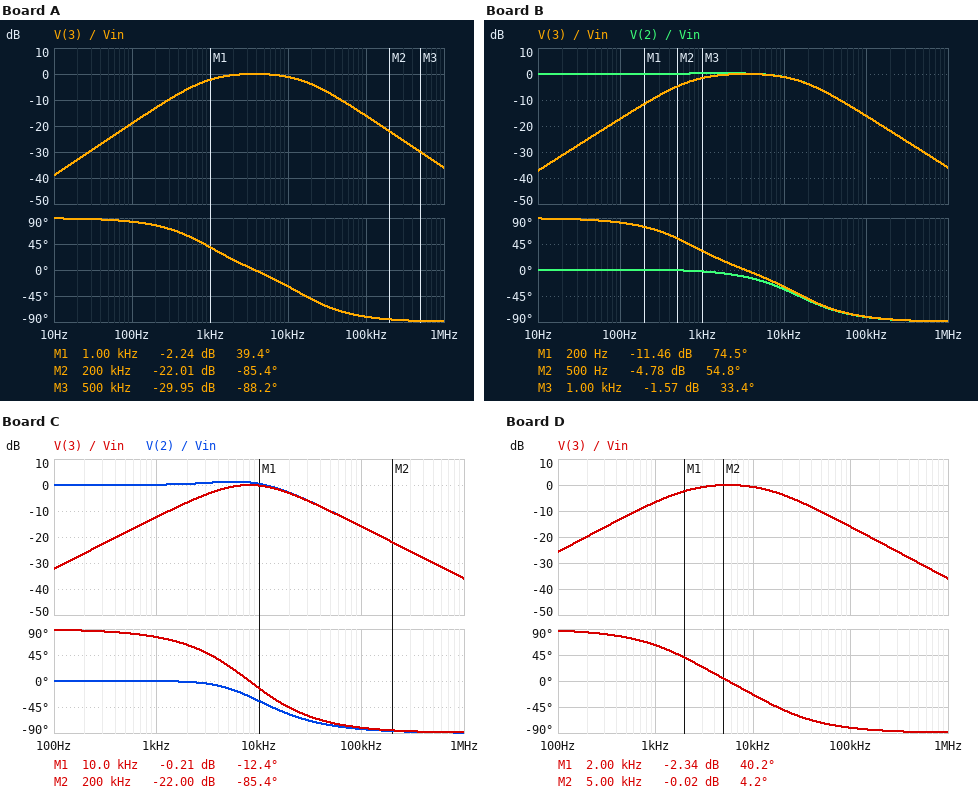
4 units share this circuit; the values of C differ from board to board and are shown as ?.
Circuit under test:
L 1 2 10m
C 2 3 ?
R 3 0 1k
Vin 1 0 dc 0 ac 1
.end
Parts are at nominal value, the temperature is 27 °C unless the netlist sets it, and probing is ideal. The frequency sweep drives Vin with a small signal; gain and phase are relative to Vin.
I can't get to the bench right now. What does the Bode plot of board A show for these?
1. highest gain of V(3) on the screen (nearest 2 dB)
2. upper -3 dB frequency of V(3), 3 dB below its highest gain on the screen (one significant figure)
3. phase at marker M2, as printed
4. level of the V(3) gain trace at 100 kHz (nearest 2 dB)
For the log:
0 dB
20 kHz
-85.4 deg
-16 dB
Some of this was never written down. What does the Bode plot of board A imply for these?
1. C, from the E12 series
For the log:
180 nF
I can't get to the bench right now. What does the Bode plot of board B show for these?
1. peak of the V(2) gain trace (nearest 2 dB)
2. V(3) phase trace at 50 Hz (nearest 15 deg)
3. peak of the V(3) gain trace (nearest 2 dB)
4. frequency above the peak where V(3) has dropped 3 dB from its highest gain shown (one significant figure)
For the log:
0 dB
90 deg
0 dB
20 kHz
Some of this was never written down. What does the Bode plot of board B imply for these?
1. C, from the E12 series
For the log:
220 nF
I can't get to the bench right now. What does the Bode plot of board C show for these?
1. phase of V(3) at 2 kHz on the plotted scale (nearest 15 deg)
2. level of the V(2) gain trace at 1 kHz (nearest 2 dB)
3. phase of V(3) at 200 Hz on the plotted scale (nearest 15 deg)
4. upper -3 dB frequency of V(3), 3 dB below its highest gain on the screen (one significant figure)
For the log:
60 deg
0 dB
90 deg
20 kHz
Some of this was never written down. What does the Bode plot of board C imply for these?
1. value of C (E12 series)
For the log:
39 nF
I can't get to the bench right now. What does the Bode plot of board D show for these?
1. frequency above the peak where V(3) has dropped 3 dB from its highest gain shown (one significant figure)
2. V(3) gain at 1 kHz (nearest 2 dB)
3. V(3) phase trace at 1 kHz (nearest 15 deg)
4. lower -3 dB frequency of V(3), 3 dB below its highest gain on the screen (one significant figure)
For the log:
20 kHz
-6 dB
60 deg
2 kHz
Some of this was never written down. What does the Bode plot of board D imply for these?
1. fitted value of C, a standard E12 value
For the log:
82 nF
